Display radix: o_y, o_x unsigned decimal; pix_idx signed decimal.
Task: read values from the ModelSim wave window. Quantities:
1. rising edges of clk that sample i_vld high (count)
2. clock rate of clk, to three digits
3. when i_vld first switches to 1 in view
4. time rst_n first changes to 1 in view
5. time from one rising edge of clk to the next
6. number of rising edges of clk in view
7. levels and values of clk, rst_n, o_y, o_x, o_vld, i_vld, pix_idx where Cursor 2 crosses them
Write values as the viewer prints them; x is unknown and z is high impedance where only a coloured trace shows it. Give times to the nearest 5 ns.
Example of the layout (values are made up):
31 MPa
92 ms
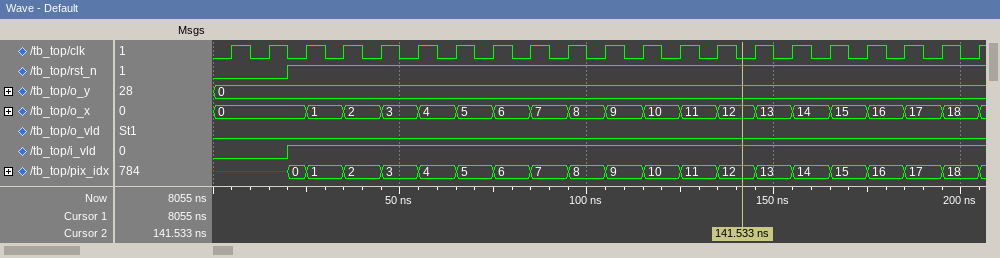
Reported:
19
100 MHz
20 ns
20 ns
10 ns
21
clk=0, rst_n=1, o_y=0, o_x=12, o_vld=0, i_vld=1, pix_idx=12
